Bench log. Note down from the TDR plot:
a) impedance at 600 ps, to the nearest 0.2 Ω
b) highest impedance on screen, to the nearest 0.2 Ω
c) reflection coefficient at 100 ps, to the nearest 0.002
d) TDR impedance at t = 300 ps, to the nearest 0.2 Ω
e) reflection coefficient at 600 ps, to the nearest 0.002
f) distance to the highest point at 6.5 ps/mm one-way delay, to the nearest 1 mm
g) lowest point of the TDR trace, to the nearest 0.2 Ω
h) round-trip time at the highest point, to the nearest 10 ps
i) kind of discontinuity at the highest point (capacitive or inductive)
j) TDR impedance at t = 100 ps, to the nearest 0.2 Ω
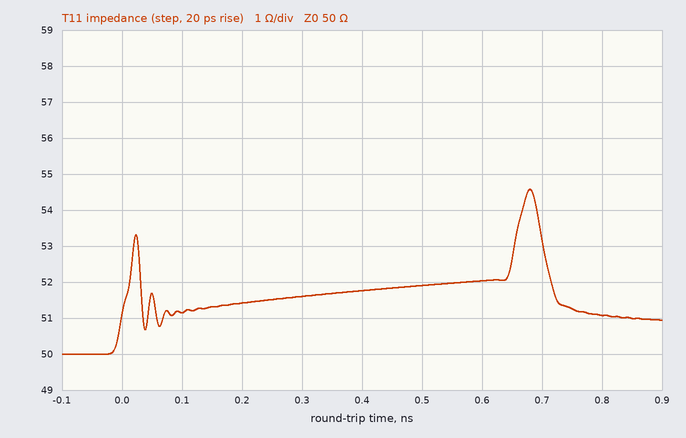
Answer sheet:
52.0 Ω
54.6 Ω
+0.012
51.6 Ω
+0.020
52 mm
50.0 Ω
680 ps
inductive
51.2 Ω
